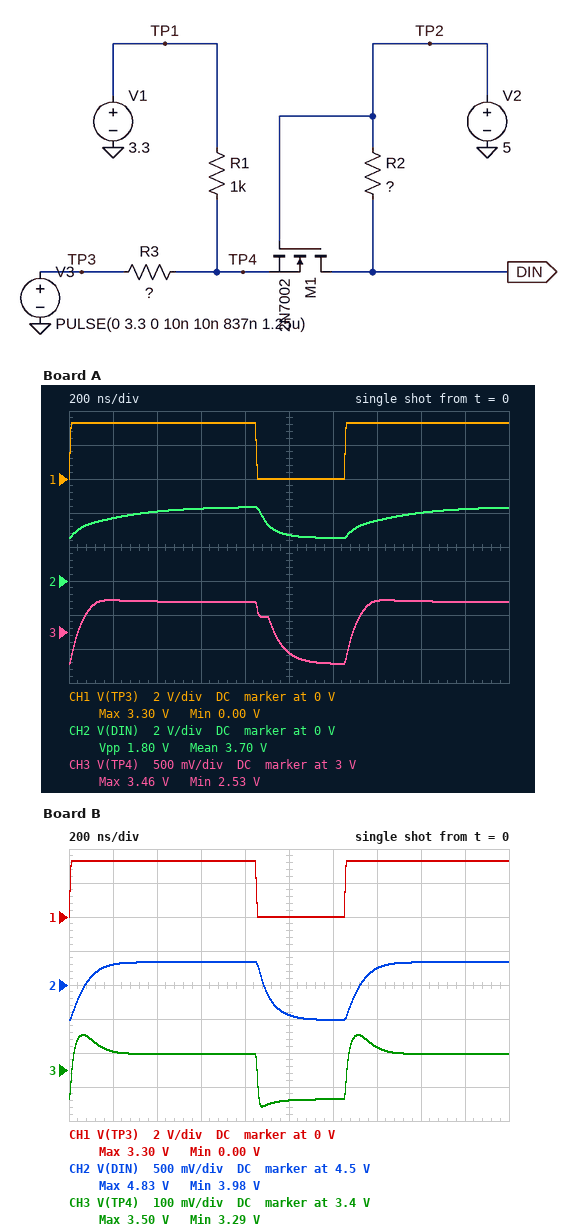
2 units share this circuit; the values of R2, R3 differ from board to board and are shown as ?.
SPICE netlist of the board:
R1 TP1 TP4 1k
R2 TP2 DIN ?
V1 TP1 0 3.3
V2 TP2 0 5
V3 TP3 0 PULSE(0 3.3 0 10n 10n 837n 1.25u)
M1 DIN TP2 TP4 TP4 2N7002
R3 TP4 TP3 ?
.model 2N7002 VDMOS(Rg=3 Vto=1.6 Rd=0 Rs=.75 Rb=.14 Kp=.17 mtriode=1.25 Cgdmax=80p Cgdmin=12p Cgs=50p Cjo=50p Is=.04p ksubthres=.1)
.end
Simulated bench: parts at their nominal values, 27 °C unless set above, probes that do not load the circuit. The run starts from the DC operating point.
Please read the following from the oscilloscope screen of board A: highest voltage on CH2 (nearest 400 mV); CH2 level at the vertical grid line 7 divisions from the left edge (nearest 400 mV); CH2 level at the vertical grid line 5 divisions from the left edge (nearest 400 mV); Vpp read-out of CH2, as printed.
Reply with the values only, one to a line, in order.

4.4 V
3.6 V
2.8 V
1.80 V
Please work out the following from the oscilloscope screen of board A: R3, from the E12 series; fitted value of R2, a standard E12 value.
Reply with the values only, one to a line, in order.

1.5 kΩ
2.7 kΩ
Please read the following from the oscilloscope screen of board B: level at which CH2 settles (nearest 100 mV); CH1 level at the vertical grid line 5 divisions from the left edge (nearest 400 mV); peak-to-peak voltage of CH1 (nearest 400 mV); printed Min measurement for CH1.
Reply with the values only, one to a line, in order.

4.8 V
0 V
3.2 V
0.00 V
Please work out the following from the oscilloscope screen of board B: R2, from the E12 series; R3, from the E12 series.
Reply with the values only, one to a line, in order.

820 Ω
2.7 kΩ
